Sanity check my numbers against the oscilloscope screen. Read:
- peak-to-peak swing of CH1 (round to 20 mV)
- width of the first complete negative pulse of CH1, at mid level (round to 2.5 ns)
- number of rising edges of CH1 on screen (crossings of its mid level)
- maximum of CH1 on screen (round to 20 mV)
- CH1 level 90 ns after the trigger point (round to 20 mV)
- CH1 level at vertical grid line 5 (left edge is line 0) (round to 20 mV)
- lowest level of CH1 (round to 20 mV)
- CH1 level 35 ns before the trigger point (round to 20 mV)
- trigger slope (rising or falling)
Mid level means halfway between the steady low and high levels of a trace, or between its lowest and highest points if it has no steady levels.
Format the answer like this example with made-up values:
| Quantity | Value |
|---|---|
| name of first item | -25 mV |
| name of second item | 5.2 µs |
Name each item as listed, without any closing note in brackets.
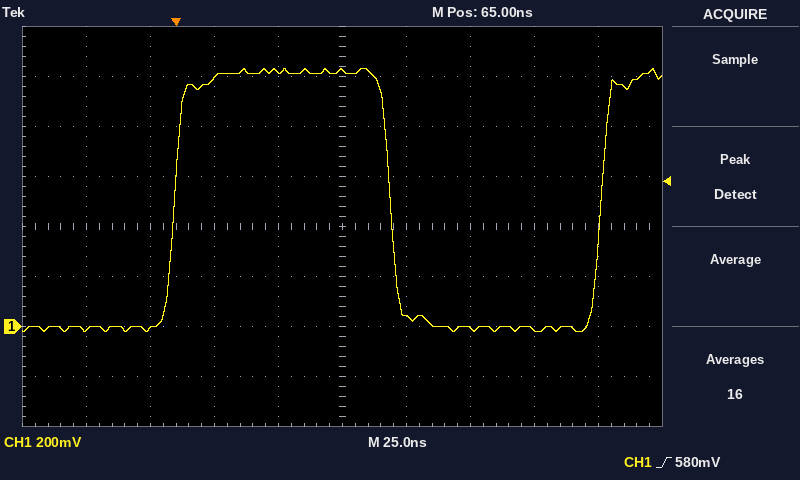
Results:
| Quantity | Value |
|---|---|
| peak-to-peak swing of CH1 | 1.06 V |
| width of the first complete negative pulse of CH1, at mid level | 82.5 ns |
| number of rising edges of CH1 on screen | 2 |
| maximum of CH1 on screen | 1.04 V |
| CH1 level 90 ns after the trigger point | 40 mV |
| CH1 level at vertical grid line 5 (left edge is line 0) | 1.02 V |
| lowest level of CH1 | -20 mV |
| CH1 level 35 ns before the trigger point | -20 mV |
| trigger slope | rising |
